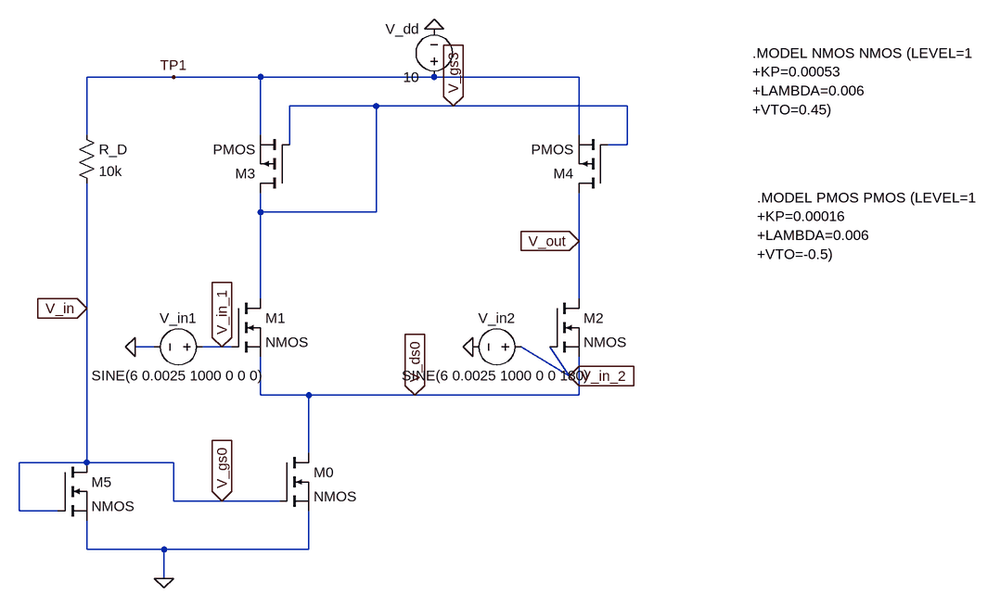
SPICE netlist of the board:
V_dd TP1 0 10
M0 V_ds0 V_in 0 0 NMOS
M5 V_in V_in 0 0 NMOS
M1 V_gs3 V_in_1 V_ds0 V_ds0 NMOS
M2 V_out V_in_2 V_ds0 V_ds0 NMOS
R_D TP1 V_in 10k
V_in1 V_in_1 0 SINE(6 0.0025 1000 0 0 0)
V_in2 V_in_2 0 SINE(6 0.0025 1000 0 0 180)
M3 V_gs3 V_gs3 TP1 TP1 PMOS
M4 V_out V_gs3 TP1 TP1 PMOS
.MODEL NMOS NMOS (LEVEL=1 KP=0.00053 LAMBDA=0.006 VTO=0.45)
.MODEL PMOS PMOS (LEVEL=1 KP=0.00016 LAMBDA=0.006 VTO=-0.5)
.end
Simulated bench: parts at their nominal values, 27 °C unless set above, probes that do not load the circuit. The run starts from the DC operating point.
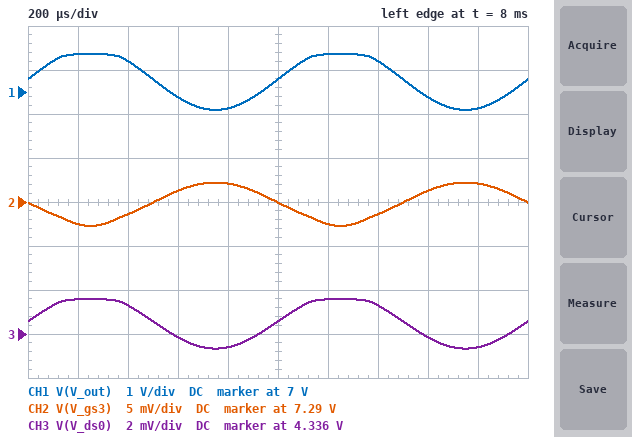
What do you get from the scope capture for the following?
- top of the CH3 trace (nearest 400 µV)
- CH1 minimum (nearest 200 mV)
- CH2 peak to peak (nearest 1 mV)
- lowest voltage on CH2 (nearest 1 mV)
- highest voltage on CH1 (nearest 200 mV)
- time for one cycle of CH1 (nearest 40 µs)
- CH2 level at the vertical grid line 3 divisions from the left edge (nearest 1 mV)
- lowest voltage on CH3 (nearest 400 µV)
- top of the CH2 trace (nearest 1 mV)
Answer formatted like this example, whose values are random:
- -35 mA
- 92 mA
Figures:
- 4.3376 V
- 6.6 V
- 5 mV
- 7.287 V
- 7.8 V
- 1.00 ms
- 7.291 V
- 4.3352 V
- 7.292 V
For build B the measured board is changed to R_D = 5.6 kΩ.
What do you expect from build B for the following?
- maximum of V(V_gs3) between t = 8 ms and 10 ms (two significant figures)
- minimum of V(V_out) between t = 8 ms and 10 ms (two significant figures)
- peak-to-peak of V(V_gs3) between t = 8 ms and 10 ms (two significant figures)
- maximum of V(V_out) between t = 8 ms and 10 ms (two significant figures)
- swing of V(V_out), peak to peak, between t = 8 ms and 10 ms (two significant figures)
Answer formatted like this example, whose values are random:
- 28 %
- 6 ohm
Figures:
- 6.7 V
- 6.1 V
- 4.6 mV
- 7.2 V
- 1.1 V
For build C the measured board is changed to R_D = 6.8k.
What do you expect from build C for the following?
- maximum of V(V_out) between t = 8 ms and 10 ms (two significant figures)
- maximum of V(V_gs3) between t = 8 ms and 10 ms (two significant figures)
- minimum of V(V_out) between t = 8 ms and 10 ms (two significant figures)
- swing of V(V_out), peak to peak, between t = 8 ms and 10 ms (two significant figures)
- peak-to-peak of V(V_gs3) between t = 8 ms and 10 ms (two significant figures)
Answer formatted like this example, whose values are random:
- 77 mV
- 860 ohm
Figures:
- 7.4 V
- 6.9 V
- 6.3 V
- 1.1 V
- 4.7 mV
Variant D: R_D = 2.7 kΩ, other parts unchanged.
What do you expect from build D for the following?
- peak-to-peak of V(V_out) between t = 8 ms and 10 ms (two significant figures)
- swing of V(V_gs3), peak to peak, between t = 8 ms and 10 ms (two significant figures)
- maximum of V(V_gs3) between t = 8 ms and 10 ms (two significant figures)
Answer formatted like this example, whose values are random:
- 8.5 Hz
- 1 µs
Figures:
- 600 mV
- 3.4 mV
- 5.7 V
